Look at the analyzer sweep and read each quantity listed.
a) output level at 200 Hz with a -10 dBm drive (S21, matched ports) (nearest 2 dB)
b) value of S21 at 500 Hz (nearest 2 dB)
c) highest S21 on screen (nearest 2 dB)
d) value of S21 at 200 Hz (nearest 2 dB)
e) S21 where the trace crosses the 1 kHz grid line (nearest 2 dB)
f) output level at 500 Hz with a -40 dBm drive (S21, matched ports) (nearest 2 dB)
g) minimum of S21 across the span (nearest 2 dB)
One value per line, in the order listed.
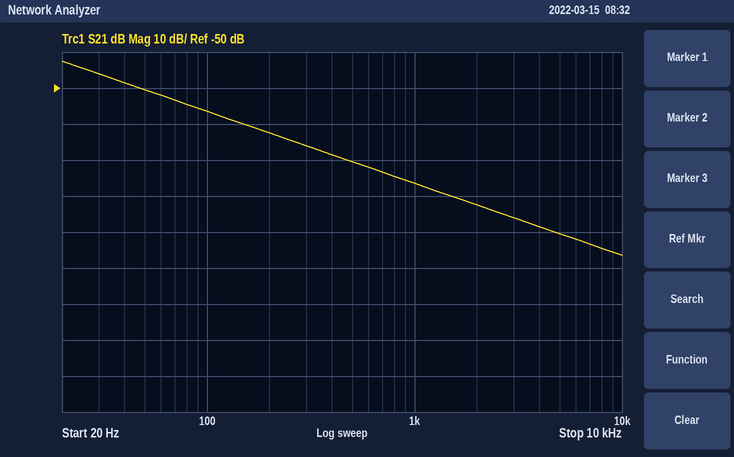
-72 dBm
-70 dB
-42 dB
-62 dB
-76 dB
-110 dBm
-96 dB
